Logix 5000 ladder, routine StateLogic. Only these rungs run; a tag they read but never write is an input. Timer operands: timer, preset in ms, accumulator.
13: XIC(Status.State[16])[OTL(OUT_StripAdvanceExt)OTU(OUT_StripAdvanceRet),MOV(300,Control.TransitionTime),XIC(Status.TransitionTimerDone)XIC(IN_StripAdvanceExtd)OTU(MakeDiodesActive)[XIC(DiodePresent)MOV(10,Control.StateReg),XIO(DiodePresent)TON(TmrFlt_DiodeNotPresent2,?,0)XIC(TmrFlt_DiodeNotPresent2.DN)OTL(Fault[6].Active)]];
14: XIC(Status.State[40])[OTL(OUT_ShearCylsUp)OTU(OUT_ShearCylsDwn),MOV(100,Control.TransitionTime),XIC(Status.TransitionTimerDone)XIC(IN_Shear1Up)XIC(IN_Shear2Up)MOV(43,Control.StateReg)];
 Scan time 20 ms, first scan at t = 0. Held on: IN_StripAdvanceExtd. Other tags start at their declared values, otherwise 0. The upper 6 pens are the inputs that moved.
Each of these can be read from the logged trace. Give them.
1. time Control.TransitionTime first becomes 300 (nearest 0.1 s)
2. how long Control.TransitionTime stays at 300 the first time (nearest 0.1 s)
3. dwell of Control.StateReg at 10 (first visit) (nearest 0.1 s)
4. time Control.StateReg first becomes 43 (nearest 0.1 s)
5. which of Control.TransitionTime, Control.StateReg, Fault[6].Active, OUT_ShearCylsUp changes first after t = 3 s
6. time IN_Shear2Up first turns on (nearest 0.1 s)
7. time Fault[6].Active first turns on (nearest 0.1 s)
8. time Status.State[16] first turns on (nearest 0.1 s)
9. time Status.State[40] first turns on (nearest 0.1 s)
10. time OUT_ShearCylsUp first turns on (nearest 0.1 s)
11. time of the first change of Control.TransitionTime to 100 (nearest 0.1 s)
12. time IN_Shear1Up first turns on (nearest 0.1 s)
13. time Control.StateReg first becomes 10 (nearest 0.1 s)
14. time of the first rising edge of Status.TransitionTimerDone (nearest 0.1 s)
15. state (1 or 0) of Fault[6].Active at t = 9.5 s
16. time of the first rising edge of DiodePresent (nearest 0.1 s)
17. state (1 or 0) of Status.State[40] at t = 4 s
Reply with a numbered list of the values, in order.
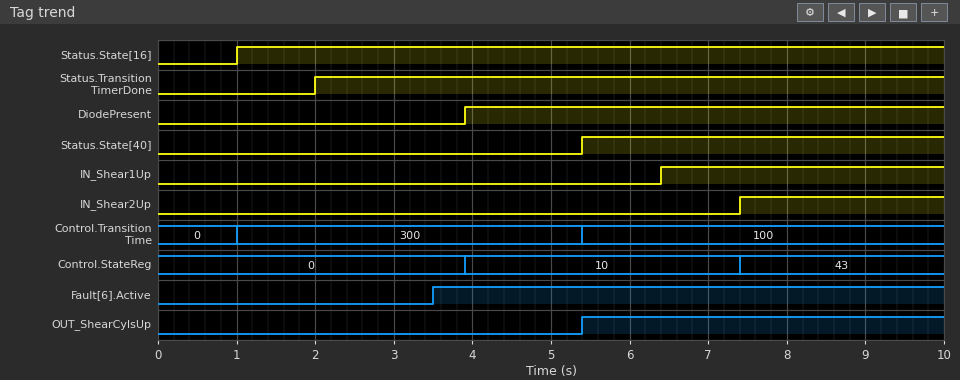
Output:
1. 1.0 s
2. 4.4 s
3. 3.5 s
4. 7.4 s
5. Fault[6].Active
6. 7.4 s
7. 3.5 s
8. 1.0 s
9. 5.4 s
10. 5.4 s
11. 5.4 s
12. 6.4 s
13. 3.9 s
14. 2.0 s
15. 1
16. 3.9 s
17. 0
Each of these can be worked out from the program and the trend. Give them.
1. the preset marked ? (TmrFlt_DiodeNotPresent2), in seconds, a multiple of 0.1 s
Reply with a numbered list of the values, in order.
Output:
1. 1.5 s
